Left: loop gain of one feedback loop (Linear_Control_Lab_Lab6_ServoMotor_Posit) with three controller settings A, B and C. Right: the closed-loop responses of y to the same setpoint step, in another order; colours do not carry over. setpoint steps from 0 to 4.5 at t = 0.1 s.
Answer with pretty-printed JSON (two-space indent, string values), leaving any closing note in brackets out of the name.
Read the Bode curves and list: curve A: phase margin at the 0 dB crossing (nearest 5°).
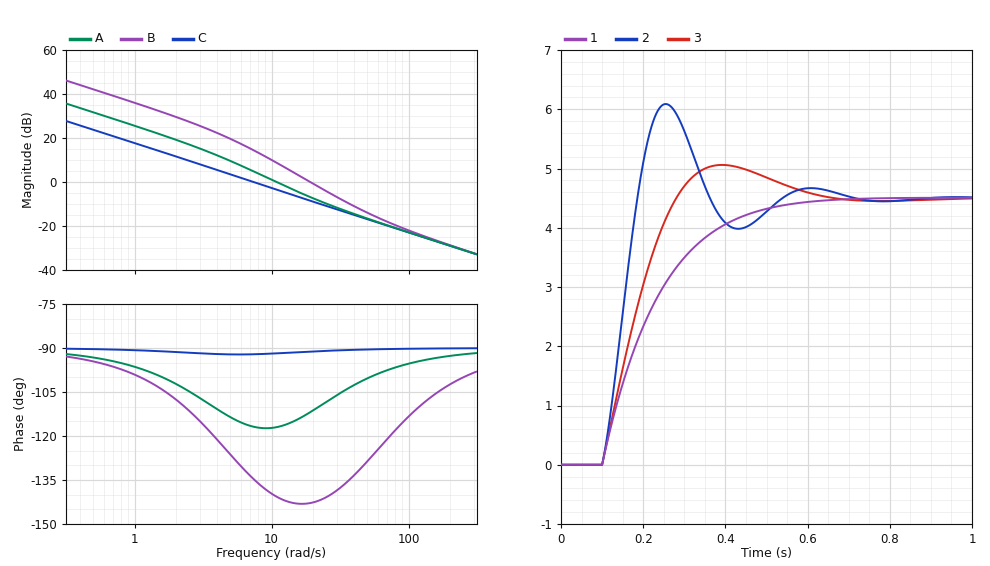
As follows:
{
  "curve A: phase margin at the 0 dB crossing": "65°"
}
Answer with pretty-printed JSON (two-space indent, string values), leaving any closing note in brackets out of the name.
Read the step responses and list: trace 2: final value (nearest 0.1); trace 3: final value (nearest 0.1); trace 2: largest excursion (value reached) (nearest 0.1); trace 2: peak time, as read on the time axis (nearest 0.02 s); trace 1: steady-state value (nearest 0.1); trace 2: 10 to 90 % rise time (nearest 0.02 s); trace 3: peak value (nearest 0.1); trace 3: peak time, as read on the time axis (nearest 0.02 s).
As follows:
{
  "trace 2: final value": "4.5",
  "trace 3: final value": "4.5",
  "trace 2: largest excursion (value reached)": "6.1",
  "trace 2: peak time, as read on the time axis": "0.26 s",
  "trace 1: steady-state value": "4.5",
  "trace 2: 10 to 90 % rise time": "0.06 s",
  "trace 3: peak value": "5.1",
  "trace 3: peak time, as read on the time axis": "0.40 s"
}
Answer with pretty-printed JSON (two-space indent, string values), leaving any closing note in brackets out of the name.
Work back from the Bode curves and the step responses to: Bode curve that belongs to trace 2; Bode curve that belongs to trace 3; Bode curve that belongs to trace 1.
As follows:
{
  "Bode curve that belongs to trace 2": "B",
  "Bode curve that belongs to trace 3": "A",
  "Bode curve that belongs to trace 1": "C"
}
